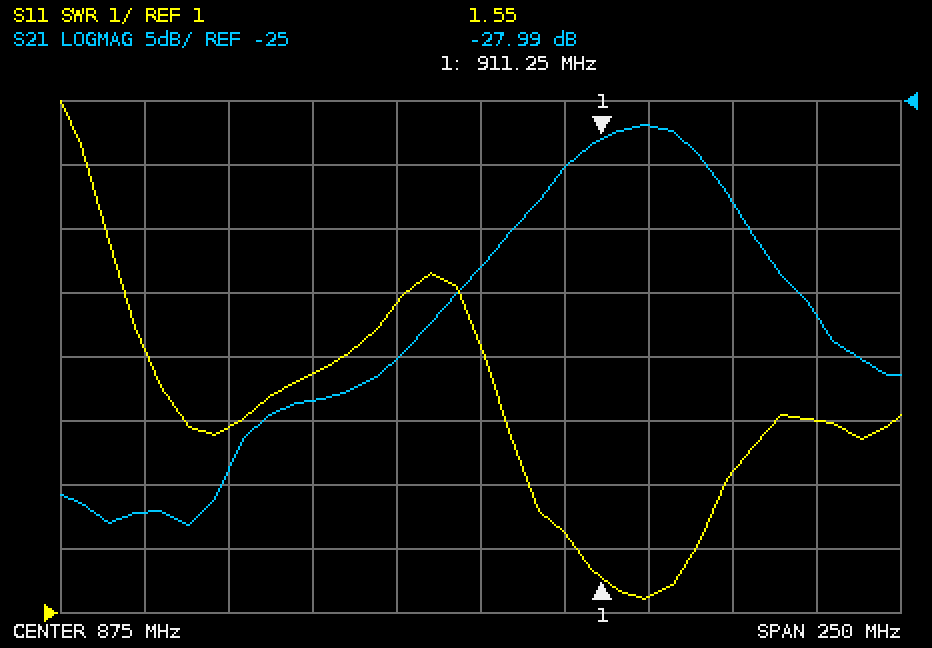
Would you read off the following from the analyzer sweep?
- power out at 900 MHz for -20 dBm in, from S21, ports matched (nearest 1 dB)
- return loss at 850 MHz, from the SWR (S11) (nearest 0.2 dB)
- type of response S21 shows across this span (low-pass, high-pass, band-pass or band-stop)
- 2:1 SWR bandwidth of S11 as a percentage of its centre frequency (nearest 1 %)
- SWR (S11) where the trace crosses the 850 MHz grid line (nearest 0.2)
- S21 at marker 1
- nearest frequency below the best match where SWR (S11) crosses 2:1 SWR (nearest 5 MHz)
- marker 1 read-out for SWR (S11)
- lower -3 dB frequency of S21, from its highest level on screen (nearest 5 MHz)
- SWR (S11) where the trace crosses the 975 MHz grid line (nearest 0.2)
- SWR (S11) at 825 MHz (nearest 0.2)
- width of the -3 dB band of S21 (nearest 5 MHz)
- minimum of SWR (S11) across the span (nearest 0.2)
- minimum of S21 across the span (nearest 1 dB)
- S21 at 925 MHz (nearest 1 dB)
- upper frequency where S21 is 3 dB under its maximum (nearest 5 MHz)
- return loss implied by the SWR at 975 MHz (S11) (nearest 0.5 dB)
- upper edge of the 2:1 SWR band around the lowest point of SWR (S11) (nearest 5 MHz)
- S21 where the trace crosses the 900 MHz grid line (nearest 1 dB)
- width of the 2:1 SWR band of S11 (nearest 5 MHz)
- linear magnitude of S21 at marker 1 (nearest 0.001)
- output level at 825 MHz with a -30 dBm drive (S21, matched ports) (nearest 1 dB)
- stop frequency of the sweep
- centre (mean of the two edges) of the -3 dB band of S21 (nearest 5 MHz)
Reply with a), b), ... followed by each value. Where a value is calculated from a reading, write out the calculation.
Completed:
a) -20 dBm + (-30 dB) = -50 dBm
b) −20 log10((5.8 − 1)/(5.8 + 1)) ≈ 3.0 dB
c) band-pass
d) 35 MHz / 922.5 MHz ≈ 4 %
e) 5.8
f) -27.99 dB
g) 905 MHz
h) 1.55
i) 900 MHz
j) 4.0
k) 4.8
l) 940 MHz − 900 MHz = 40 MHz
m) 1.2
n) -58 dB
o) -27 dB
p) 940 MHz
q) −20 log10((4 − 1)/(4 + 1)) ≈ 4.44 dB, so 4.5 dB to the nearest 0.5 dB
r) 940 MHz
s) -30 dB
t) 940 MHz − 905 MHz = 35 MHz
u) 10^(-27.99/20) ≈ 0.040
v) -30 dBm + (-48 dB) = -78 dBm
w) 1 GHz
x) 920 MHz
